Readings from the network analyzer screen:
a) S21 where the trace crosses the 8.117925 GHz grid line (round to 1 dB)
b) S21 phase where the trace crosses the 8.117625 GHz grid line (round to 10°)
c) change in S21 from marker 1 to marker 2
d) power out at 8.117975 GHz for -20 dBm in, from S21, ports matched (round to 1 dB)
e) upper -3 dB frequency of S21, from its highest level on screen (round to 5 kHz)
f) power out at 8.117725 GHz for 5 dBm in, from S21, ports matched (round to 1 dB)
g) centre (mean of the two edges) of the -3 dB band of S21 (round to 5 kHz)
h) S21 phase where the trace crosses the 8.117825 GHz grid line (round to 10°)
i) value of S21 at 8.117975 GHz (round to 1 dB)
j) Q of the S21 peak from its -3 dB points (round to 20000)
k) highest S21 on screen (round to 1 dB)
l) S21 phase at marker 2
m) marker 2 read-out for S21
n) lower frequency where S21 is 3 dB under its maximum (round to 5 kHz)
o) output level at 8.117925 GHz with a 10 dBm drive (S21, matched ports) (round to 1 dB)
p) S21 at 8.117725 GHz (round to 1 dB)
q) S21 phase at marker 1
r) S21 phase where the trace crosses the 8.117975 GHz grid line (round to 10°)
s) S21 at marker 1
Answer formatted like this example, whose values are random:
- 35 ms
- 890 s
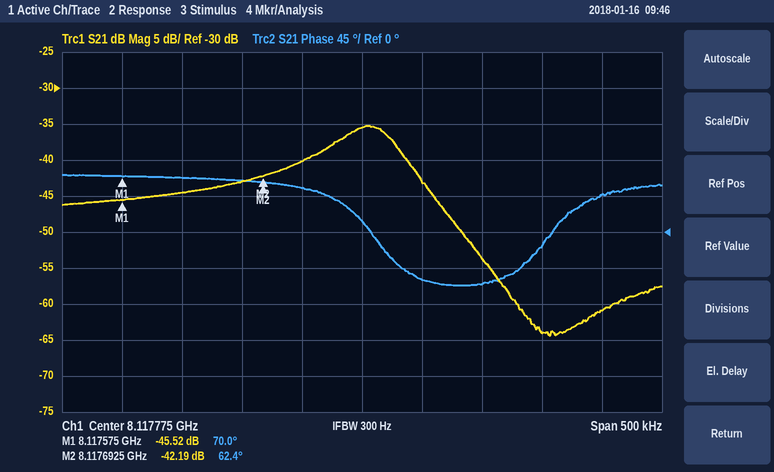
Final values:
- -64 dB
- 70°
- 3.33 dB
- -81 dBm
- 8.117805 GHz
- -35 dBm
- 8.117775 GHz
- -60°
- -61 dB
- 140000
- -35 dB
- 62.4°
- -42.19 dB
- 8.117745 GHz
- -54 dBm
- -40 dB
- 70.0°
- 50°
- -45.52 dB
